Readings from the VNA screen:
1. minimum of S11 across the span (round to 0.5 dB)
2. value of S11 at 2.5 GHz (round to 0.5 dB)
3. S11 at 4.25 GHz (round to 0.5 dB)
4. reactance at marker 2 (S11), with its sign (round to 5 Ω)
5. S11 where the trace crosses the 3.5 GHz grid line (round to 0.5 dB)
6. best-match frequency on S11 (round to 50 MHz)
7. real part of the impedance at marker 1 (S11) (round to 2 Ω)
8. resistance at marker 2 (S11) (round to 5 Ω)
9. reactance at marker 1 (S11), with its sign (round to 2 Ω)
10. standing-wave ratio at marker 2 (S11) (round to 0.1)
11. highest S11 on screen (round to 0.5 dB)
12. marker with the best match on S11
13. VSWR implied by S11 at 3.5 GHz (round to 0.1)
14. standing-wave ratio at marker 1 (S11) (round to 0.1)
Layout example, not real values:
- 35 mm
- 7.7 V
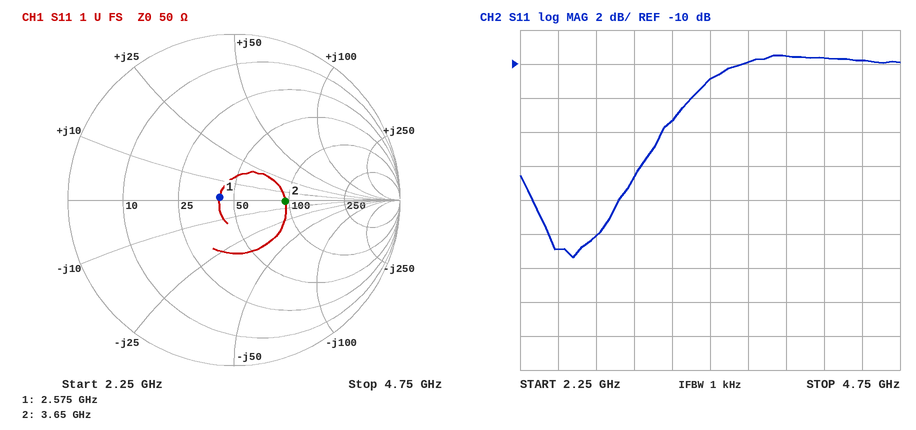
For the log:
- -21.5 dB
- -21.0 dB
- -9.5 dB
- 0 Ω
- -11.0 dB
- 2.60 GHz
- 42 Ω
- 95 Ω
- +2 Ω
- 1.9
- -9.5 dB
- marker 1
- 1.8
- 1.2
